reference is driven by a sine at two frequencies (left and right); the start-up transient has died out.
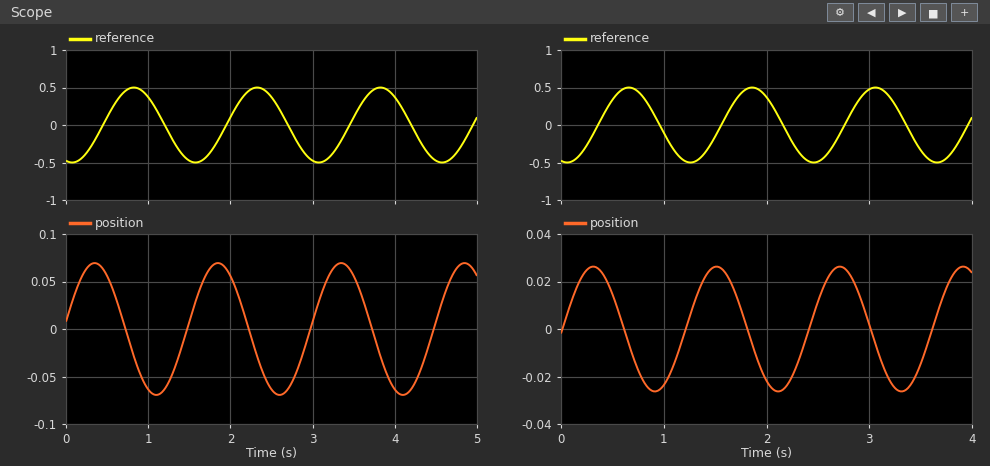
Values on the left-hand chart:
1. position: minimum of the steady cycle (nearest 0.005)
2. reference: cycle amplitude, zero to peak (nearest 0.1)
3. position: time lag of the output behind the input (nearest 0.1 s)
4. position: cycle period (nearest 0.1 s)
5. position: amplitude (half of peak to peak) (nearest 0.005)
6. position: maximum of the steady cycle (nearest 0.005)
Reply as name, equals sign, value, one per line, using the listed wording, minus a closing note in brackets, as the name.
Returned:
position: minimum of the steady cycle = -0.070
reference: cycle amplitude, zero to peak = 0.5
position: time lag of the output behind the input = 1.0 s
position: cycle period = 1.5 s
position: amplitude (half of peak to peak) = 0.070
position: maximum of the steady cycle = 0.070
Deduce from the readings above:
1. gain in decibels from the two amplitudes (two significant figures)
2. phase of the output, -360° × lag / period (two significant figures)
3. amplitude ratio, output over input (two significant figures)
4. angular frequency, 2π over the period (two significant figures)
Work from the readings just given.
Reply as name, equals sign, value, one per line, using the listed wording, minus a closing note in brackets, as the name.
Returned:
gain in decibels from the two amplitudes = -17 dB
phase of the output, -360° × lag / period = -240°
amplitude ratio, output over input = 0.14
angular frequency, 2π over the period = 4.2 rad/s
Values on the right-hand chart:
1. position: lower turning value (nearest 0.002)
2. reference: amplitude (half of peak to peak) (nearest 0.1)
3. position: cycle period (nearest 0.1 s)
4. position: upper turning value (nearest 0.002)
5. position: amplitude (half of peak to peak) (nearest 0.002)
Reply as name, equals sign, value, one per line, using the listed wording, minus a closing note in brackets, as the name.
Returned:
position: lower turning value = -0.026
reference: amplitude (half of peak to peak) = 0.5
position: cycle period = 1.2 s
position: upper turning value = 0.026
position: amplitude (half of peak to peak) = 0.026
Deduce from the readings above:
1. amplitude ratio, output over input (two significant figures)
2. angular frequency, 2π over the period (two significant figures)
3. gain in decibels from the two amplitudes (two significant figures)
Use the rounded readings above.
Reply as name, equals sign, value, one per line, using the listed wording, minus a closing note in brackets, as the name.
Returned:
amplitude ratio, output over input = 0.052
angular frequency, 2π over the period = 5.2 rad/s
gain in decibels from the two amplitudes = -26 dB
